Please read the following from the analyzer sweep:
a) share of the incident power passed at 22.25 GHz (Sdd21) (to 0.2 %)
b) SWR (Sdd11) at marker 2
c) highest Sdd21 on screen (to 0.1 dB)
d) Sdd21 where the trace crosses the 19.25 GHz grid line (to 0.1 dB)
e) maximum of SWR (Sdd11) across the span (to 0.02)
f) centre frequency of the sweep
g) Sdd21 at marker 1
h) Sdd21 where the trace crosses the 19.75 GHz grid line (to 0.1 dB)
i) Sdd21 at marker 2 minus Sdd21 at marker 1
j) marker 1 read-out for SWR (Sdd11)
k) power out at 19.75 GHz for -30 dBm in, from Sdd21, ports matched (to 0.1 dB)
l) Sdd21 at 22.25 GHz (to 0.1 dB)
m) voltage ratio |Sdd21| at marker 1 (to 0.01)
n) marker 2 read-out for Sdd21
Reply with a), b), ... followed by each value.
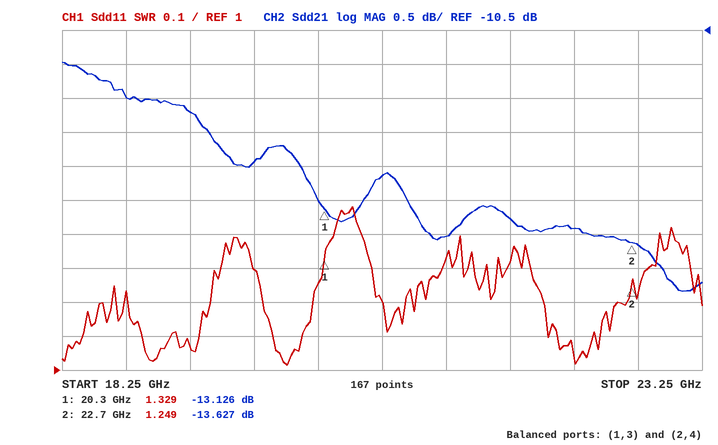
a) 4.6 %
b) 1.249
c) -11.0 dB
d) -11.7 dB
e) 1.48
f) 20.75 GHz
g) -13.126 dB
h) -12.4 dB
i) -0.501 dB
j) 1.329
k) -42.4 dBm
l) -13.4 dB
m) 0.22
n) -13.627 dB
